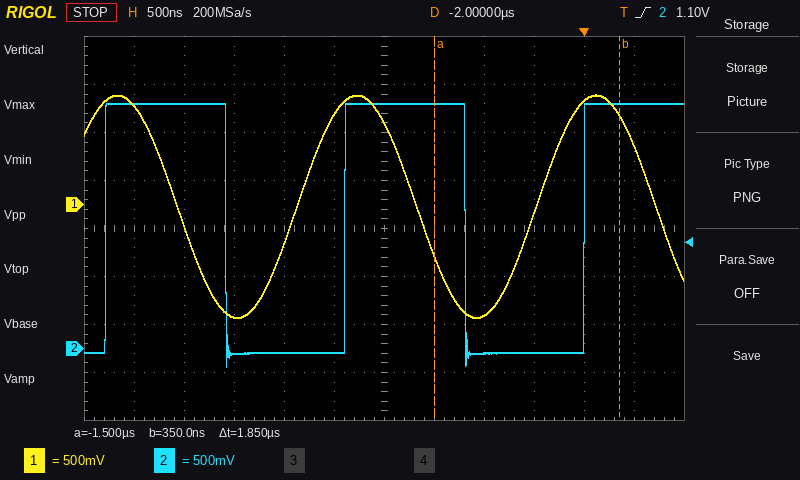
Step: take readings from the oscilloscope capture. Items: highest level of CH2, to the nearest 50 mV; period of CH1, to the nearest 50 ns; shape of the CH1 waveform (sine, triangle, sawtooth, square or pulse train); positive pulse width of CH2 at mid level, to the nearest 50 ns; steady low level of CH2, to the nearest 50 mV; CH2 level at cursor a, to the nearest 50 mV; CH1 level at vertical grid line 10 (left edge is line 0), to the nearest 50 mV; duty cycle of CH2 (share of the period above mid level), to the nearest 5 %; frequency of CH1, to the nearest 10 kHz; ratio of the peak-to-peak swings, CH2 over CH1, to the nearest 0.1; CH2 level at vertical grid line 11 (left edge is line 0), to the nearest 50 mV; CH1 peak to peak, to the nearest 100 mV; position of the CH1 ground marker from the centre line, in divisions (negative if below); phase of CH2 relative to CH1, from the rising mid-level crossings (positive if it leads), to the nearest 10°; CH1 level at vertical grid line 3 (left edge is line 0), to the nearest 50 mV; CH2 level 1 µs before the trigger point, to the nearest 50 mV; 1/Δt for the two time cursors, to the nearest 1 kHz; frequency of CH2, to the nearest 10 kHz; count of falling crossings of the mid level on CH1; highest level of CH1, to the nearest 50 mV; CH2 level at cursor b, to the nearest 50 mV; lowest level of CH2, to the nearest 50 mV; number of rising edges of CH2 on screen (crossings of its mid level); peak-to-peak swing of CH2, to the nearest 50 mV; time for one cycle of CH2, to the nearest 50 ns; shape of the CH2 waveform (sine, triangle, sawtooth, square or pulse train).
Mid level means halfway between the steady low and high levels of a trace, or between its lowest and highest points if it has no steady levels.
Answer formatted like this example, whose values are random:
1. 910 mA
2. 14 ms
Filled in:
1. 2.55 V
2. 2.40 µs
3. sine
4. 1.20 µs
5. -50 mV
6. 2.55 V
7. 1.10 V
8. 50 %
9. 420 kHz
10. 1.2
11. 2.55 V
12. 2.30 V
13. +0.5 div
14. -70°
15. -1.15 V
16. -50 mV
17. 541 kHz
18. 420 kHz
19. 3
20. 1.15 V
21. 2.55 V
22. -200 mV
23. 3
24. 2.75 V
25. 2.40 µs
26. square
